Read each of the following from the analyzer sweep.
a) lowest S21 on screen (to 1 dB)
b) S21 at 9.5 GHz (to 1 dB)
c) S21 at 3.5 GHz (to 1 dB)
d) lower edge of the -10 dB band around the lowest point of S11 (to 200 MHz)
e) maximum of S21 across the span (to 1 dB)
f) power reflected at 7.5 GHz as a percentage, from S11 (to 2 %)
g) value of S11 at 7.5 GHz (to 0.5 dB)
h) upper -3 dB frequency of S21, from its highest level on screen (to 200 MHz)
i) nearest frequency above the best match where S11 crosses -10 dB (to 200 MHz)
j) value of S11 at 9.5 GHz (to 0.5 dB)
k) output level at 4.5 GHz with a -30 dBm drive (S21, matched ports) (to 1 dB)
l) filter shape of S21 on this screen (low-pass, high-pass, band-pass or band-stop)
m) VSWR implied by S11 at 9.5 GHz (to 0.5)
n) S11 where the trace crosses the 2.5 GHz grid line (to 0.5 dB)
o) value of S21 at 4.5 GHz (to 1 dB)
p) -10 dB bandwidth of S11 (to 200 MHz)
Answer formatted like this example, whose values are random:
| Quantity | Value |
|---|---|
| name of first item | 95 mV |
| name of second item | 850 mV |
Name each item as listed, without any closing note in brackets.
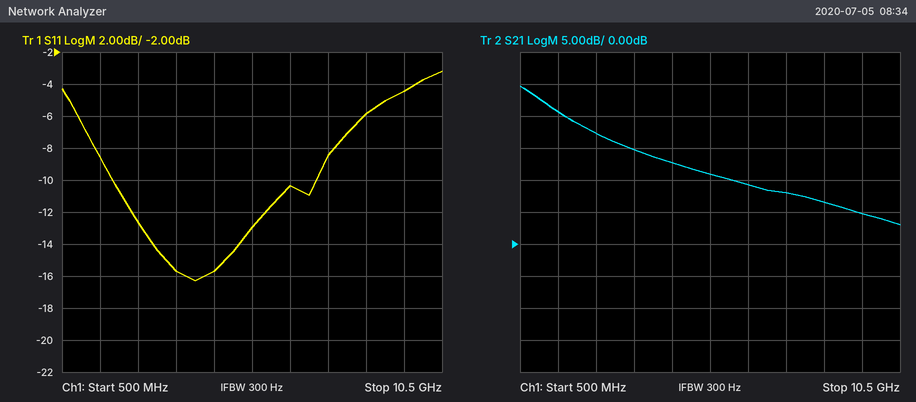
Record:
| Quantity | Value |
|---|---|
| lowest S21 on screen | 3 dB |
| S21 at 9.5 GHz | 5 dB |
| S21 at 3.5 GHz | 15 dB |
| lower edge of the -10 dB band around the lowest point of S11 | 1.8 GHz |
| maximum of S21 across the span | 25 dB |
| power reflected at 7.5 GHz as a percentage, from S11 | 14 % |
| value of S11 at 7.5 GHz | -8.5 dB |
| upper -3 dB frequency of S21, from its highest level on screen | 1.2 GHz |
| nearest frequency above the best match where S11 crosses -10 dB | 7.2 GHz |
| value of S11 at 9.5 GHz | -4.5 dB |
| output level at 4.5 GHz with a -30 dBm drive (S21, matched ports) | -17 dBm |
| filter shape of S21 on this screen | low-pass |
| VSWR implied by S11 at 9.5 GHz | 4.0 |
| S11 where the trace crosses the 2.5 GHz grid line | -12.5 dB |
| value of S21 at 4.5 GHz | 13 dB |
| -10 dB bandwidth of S11 | 5.4 GHz |
